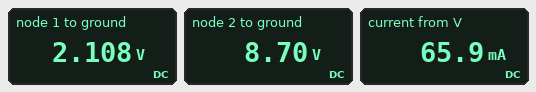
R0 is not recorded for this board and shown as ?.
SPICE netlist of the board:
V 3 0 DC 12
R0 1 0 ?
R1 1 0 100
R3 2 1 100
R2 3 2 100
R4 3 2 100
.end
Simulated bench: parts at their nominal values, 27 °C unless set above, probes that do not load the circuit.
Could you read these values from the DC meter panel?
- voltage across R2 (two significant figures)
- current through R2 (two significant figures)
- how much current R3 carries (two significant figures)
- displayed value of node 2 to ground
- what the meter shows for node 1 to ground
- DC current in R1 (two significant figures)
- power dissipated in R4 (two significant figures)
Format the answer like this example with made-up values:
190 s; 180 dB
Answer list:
3.3 V; 33 mA; 66 mA; 8.70 V; 2.108 V; 21 mA; 110 mW
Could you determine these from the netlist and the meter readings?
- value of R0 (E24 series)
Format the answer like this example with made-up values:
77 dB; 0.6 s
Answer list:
47 Ω
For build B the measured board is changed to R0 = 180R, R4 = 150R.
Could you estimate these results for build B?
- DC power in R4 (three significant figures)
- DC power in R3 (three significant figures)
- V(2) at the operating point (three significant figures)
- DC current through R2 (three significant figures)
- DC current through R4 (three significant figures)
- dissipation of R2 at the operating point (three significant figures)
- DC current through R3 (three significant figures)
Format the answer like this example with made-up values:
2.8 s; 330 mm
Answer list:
68.7 mW; 286 mW; 8.79 V; 32.1 mA; 21.4 mA; 103 mW; 53.5 mA
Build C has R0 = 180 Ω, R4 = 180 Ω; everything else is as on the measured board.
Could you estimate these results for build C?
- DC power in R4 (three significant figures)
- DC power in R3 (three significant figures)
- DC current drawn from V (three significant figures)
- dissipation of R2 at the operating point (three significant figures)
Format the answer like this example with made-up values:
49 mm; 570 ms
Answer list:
63.3 mW; 276 mW; 52.5 mA; 114 mW
